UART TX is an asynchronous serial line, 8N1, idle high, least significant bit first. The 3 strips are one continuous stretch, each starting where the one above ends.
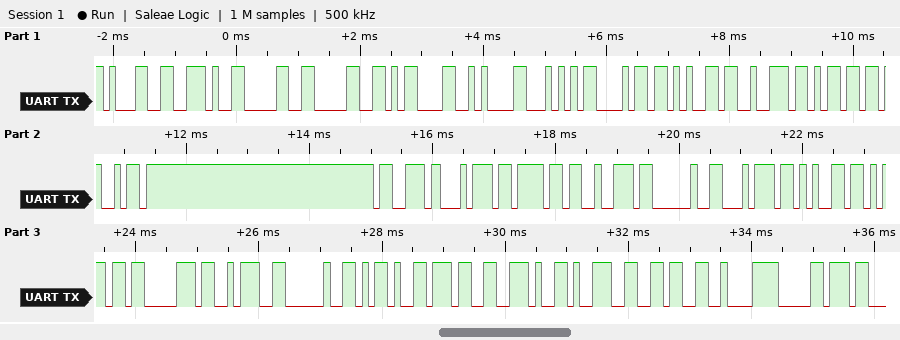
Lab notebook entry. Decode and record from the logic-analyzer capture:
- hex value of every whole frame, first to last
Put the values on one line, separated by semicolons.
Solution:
31 2E 30 30 0D 0A 54 68 65 72 6D 69 73 74 6F 72 20 74 65 6D 70 3A 20 2D 37 2E 39 36 C2 B0
